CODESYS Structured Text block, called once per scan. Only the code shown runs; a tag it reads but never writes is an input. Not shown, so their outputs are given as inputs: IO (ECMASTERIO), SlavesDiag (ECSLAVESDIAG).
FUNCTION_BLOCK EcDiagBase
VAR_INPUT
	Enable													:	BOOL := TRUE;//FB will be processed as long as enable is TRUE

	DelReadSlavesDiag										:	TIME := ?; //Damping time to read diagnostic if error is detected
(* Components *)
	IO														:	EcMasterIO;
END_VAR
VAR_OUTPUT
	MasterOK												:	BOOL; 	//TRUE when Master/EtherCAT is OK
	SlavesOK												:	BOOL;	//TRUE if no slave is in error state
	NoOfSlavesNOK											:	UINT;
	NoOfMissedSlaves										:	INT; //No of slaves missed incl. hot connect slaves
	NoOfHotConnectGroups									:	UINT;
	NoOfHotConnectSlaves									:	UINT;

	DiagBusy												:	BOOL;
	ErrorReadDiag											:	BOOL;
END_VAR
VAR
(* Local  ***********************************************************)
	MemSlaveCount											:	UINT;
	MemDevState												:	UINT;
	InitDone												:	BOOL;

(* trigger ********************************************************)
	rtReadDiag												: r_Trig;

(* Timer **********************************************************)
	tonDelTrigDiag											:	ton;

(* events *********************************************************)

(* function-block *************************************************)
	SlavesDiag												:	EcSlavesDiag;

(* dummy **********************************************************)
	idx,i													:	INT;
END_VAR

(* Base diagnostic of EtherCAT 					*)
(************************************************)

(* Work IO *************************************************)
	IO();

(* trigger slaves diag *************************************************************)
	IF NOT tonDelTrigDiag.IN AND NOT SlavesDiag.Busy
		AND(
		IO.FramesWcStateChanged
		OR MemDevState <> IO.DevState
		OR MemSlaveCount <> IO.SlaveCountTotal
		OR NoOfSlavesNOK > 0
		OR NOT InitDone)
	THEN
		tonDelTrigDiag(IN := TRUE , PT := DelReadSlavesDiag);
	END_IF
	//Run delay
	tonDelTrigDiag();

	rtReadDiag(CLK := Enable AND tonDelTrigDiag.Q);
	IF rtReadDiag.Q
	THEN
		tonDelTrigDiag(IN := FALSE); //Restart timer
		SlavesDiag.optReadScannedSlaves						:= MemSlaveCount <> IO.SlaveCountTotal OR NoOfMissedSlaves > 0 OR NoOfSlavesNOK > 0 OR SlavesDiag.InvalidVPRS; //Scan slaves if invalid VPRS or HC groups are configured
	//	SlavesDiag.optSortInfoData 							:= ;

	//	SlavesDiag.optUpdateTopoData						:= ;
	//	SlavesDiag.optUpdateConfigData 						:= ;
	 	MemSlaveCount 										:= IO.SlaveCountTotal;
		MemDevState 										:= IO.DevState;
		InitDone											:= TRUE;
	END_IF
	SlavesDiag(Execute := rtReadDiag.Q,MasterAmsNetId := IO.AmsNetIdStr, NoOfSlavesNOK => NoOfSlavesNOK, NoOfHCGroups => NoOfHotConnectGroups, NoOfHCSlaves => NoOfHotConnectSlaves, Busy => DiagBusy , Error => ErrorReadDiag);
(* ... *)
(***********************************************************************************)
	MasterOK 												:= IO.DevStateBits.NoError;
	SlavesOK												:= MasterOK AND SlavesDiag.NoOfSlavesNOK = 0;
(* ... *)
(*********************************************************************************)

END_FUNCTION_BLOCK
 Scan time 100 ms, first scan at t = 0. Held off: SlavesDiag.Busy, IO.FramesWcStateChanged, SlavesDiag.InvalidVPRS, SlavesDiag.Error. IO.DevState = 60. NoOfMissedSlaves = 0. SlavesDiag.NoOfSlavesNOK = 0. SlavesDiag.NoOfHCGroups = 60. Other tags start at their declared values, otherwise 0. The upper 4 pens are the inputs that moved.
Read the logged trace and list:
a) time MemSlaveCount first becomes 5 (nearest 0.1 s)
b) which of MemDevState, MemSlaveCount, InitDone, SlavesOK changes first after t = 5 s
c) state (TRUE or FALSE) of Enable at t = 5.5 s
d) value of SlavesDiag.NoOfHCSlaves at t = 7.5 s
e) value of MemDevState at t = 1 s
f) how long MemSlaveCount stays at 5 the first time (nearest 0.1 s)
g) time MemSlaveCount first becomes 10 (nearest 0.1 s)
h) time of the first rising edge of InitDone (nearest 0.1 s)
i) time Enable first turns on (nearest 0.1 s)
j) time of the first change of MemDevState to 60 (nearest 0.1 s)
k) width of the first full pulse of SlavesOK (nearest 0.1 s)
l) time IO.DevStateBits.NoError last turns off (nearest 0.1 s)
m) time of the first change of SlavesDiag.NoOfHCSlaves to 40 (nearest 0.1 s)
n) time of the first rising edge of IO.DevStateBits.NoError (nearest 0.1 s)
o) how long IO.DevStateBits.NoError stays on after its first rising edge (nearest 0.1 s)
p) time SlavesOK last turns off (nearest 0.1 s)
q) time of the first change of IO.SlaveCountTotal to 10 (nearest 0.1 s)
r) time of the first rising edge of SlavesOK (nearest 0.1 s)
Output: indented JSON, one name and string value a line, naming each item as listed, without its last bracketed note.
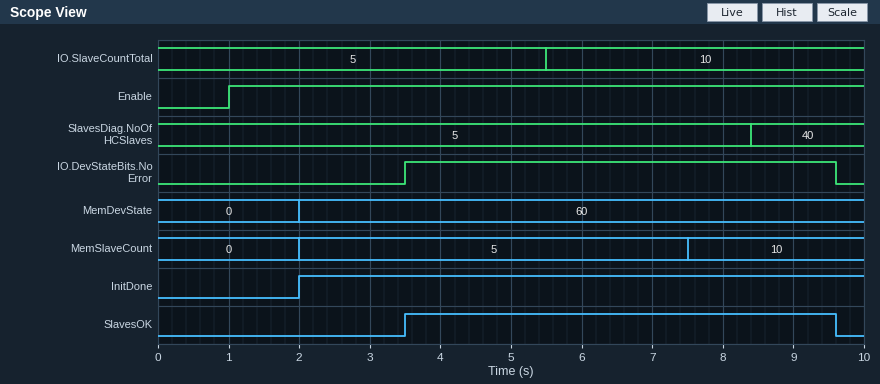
{
  "time MemSlaveCount first becomes 5": "2.0 s",
  "which of MemDevState, MemSlaveCount, InitDone, SlavesOK changes first after t = 5 s": "MemSlaveCount",
  "state (TRUE or FALSE) of Enable at t = 5.5 s": "TRUE",
  "value of SlavesDiag.NoOfHCSlaves at t = 7.5 s": "5",
  "value of MemDevState at t = 1 s": "0",
  "how long MemSlaveCount stays at 5 the first time": "5.5 s",
  "time MemSlaveCount first becomes 10": "7.5 s",
  "time of the first rising edge of InitDone": "2.0 s",
  "time Enable first turns on": "1.0 s",
  "time of the first change of MemDevState to 60": "2.0 s",
  "width of the first full pulse of SlavesOK": "6.1 s",
  "time IO.DevStateBits.NoError last turns off": "9.6 s",
  "time of the first change of SlavesDiag.NoOfHCSlaves to 40": "8.4 s",
  "time of the first rising edge of IO.DevStateBits.NoError": "3.5 s",
  "how long IO.DevStateBits.NoError stays on after its first rising edge": "6.1 s",
  "time SlavesOK last turns off": "9.6 s",
  "time of the first change of IO.SlaveCountTotal to 10": "5.5 s",
  "time of the first rising edge of SlavesOK": "3.5 s"
}
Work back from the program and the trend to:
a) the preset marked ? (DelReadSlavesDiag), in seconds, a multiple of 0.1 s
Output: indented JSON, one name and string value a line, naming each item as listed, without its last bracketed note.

{
  "the preset marked ? (DelReadSlavesDiag), in seconds, a multiple of 0.1 s": "2.0 s"
}
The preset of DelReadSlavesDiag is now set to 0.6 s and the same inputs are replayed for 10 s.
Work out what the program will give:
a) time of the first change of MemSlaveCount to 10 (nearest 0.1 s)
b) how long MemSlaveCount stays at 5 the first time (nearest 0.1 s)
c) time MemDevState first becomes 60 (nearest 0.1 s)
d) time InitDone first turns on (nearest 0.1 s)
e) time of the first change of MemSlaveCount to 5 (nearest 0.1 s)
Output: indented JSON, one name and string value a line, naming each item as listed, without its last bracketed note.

{
  "time of the first change of MemSlaveCount to 10": "6.1 s",
  "how long MemSlaveCount stays at 5 the first time": "5.1 s",
  "time MemDevState first becomes 60": "1.0 s",
  "time InitDone first turns on": "1.0 s",
  "time of the first change of MemSlaveCount to 5": "1.0 s"
}
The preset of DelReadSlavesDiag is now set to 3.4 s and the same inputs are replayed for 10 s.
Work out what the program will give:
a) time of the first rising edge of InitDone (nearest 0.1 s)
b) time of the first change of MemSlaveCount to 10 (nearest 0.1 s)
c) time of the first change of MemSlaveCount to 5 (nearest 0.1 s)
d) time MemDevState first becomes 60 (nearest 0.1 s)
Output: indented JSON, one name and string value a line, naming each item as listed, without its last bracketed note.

{
  "time of the first rising edge of InitDone": "3.4 s",
  "time of the first change of MemSlaveCount to 10": "8.9 s",
  "time of the first change of MemSlaveCount to 5": "3.4 s",
  "time MemDevState first becomes 60": "3.4 s"
}
